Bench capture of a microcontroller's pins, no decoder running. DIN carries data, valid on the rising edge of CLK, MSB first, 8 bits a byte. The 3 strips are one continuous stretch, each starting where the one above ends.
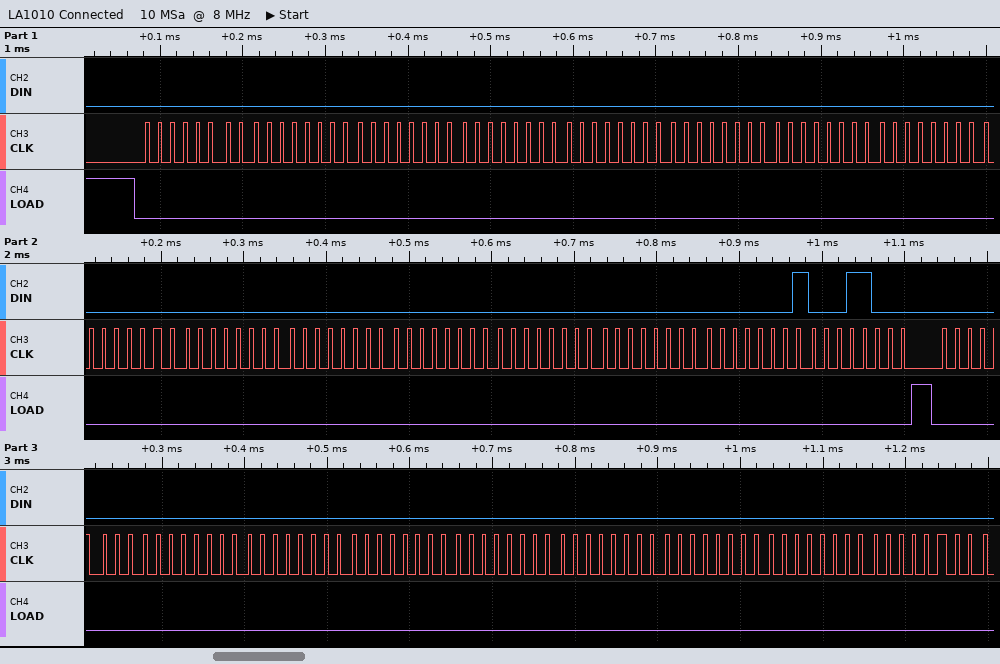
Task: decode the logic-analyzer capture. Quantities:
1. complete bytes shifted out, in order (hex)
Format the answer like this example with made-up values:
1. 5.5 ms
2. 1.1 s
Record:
1. 0x00 0x00 0x00 0x00 0x00 0x00 0x00 0x00 0x00 0x00 0x00 0x00 0x00 0x00 0x01 0x18 0x00 0x00 0x00 0x00 0x00 0x00 0x00 0x00 0x00
